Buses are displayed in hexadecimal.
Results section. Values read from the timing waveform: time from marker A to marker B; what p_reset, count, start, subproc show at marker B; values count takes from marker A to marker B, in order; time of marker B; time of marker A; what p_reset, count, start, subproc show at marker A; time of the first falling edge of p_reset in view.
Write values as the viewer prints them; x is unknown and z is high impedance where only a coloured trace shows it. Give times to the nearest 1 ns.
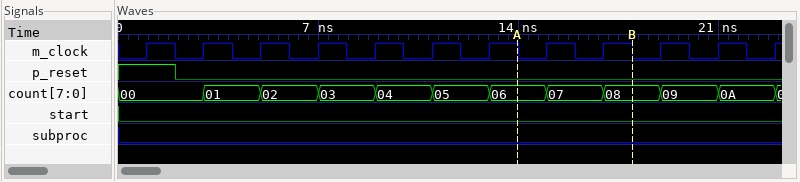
4 ns
p_reset=0, count=08, start=0, subproc=0
06, 07, 08
18 ns
14 ns
p_reset=0, count=06, start=0, subproc=0
2 ns
